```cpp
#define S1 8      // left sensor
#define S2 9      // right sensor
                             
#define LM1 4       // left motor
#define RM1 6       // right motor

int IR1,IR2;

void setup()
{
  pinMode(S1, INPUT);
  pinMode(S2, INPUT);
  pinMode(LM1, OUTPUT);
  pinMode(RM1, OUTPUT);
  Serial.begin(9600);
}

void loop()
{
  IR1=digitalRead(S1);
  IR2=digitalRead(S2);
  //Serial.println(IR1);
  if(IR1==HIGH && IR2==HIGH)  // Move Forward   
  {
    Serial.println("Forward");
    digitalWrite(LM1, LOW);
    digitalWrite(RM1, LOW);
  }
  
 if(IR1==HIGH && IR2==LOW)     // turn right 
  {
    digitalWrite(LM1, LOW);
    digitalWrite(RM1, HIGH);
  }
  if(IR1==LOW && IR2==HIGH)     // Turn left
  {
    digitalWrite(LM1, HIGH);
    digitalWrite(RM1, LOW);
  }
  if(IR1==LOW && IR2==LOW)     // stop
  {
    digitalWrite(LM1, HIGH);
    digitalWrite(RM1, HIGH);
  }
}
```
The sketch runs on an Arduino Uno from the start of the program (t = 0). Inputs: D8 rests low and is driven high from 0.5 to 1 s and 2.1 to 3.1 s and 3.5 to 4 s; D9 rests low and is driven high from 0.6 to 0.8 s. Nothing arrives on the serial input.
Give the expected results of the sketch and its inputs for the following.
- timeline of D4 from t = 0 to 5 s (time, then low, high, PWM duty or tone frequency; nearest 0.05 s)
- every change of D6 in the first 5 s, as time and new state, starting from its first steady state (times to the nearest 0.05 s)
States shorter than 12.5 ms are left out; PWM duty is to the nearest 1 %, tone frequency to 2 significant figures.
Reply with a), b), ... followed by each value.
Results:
a) 0 s high; 0.5 s low; 1 s high; 2.1 s low; 3.1 s high; 3.5 s low; 4 s high
b) 0 s high; 0.6 s low; 0.8 s high
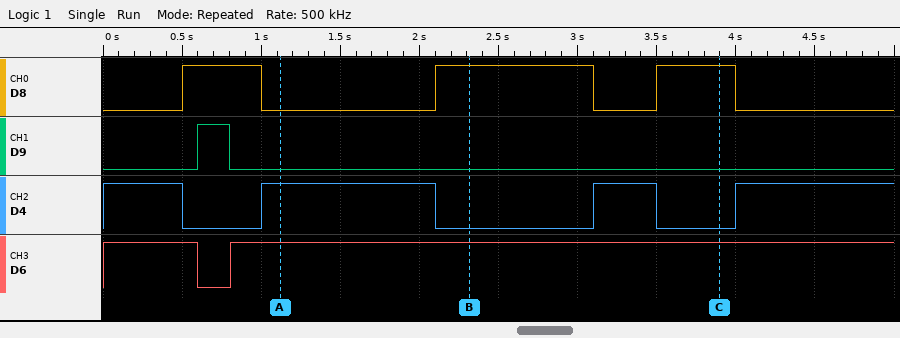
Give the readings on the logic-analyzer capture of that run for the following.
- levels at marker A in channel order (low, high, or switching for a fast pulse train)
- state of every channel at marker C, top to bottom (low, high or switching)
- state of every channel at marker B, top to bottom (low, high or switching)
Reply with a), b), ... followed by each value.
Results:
a) D8 low, D9 low, D4 high, D6 high
b) D8 high, D9 low, D4 low, D6 high
c) D8 high, D9 low, D4 low, D6 high
